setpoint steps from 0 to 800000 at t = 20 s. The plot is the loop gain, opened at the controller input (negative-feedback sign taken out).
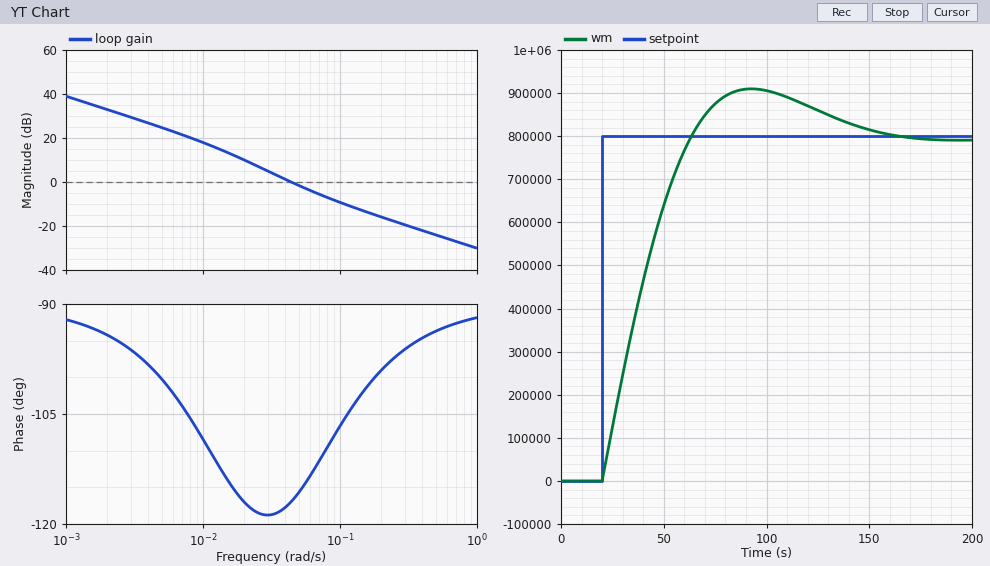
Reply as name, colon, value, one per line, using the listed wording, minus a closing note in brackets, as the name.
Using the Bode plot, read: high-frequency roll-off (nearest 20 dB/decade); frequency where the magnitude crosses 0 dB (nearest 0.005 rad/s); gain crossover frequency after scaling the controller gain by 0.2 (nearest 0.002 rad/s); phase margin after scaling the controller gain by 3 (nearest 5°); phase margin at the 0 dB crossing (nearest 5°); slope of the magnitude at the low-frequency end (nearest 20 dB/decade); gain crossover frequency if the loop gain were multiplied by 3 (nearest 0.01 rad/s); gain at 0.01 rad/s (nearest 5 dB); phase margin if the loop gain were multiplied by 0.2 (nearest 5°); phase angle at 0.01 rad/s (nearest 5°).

high-frequency roll-off: -20 dB/decade
frequency where the magnitude crosses 0 dB: 0.045 rad/s
gain crossover frequency after scaling the controller gain by 0.2: 0.014 rad/s
phase margin after scaling the controller gain by 3: 75°
phase margin at the 0 dB crossing: 65°
slope of the magnitude at the low-frequency end: -20 dB/decade
gain crossover frequency if the loop gain were multiplied by 3: 0.10 rad/s
gain at 0.01 rad/s: 20 dB
phase margin if the loop gain were multiplied by 0.2: 65°
phase angle at 0.01 rad/s: -110°
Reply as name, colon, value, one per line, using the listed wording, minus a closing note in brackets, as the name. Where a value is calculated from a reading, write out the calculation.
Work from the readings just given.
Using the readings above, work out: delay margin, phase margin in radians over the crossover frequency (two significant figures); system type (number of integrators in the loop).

delay margin, phase margin in radians over the crossover frequency: 65 × π / 180 / 0.045 = 25 s
system type: 1
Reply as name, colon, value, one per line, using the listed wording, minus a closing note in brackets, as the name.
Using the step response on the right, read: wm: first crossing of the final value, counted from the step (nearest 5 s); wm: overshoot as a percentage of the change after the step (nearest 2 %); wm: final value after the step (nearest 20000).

wm: first crossing of the final value, counted from the step: 45 s
wm: overshoot as a percentage of the change after the step: 14 %
wm: final value after the step: 800000
